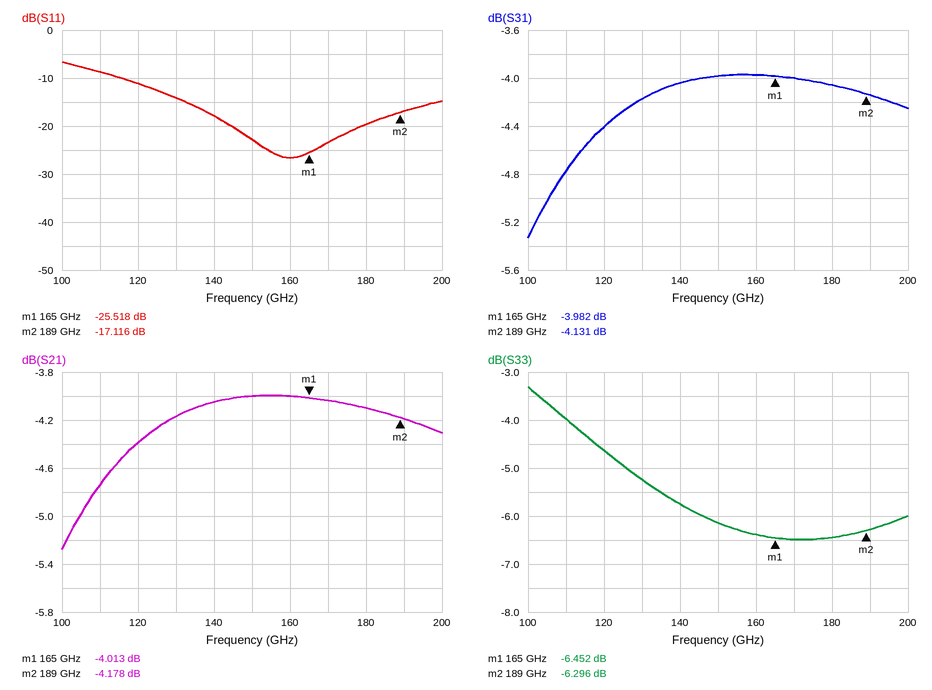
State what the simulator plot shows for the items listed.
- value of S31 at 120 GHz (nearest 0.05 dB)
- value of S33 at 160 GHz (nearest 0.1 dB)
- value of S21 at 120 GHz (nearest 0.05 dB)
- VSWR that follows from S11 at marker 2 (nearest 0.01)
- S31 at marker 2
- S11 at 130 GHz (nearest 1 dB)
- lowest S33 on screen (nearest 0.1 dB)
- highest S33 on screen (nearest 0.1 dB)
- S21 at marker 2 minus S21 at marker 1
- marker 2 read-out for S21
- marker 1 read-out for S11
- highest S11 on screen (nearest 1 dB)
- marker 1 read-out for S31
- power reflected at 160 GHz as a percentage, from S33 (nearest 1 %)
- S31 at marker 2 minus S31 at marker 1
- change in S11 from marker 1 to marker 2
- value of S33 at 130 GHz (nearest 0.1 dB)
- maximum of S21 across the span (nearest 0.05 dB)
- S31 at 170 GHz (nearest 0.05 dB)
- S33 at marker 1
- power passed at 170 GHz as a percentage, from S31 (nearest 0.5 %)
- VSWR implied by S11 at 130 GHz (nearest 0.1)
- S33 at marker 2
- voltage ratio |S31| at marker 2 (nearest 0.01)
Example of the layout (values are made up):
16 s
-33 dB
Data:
-4.40 dB
-6.4 dB
-4.40 dB
1.32
-4.131 dB
-14 dB
-6.5 dB
-3.3 dB
-0.165 dB
-4.178 dB
-25.518 dB
-7 dB
-3.982 dB
23 %
-0.149 dB
8.402 dB
-5.2 dB
-4.00 dB
-4.00 dB
-6.452 dB
40.0 %
1.5
-6.296 dB
0.62
